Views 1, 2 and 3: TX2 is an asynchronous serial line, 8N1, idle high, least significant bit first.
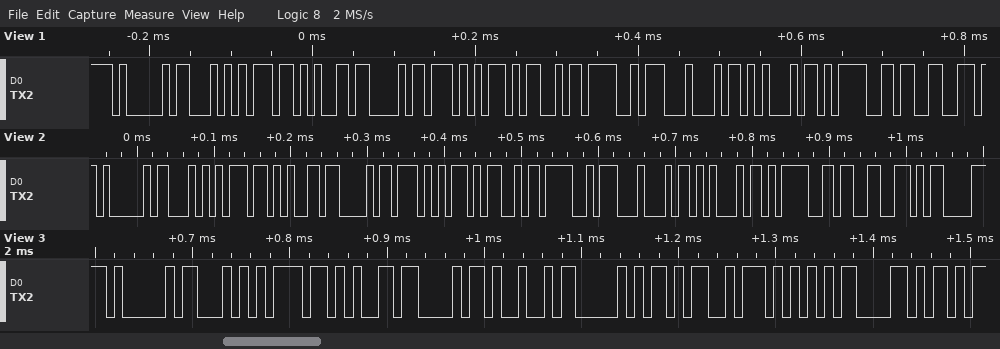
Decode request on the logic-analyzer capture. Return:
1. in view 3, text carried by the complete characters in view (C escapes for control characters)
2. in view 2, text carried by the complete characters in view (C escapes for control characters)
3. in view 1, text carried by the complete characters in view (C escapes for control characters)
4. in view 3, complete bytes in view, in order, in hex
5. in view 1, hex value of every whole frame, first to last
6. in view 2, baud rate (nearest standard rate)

"AT+CIPMUX"
"AT+CWMODE=3\r"
"AT+CWMODE=3"
0x41 0x54 0x2B 0x43 0x49 0x50 0x4D 0x55 0x58
0x41 0x54 0x2B 0x43 0x57 0x4D 0x4F 0x44 0x45 0x3D 0x33
115200 baud
